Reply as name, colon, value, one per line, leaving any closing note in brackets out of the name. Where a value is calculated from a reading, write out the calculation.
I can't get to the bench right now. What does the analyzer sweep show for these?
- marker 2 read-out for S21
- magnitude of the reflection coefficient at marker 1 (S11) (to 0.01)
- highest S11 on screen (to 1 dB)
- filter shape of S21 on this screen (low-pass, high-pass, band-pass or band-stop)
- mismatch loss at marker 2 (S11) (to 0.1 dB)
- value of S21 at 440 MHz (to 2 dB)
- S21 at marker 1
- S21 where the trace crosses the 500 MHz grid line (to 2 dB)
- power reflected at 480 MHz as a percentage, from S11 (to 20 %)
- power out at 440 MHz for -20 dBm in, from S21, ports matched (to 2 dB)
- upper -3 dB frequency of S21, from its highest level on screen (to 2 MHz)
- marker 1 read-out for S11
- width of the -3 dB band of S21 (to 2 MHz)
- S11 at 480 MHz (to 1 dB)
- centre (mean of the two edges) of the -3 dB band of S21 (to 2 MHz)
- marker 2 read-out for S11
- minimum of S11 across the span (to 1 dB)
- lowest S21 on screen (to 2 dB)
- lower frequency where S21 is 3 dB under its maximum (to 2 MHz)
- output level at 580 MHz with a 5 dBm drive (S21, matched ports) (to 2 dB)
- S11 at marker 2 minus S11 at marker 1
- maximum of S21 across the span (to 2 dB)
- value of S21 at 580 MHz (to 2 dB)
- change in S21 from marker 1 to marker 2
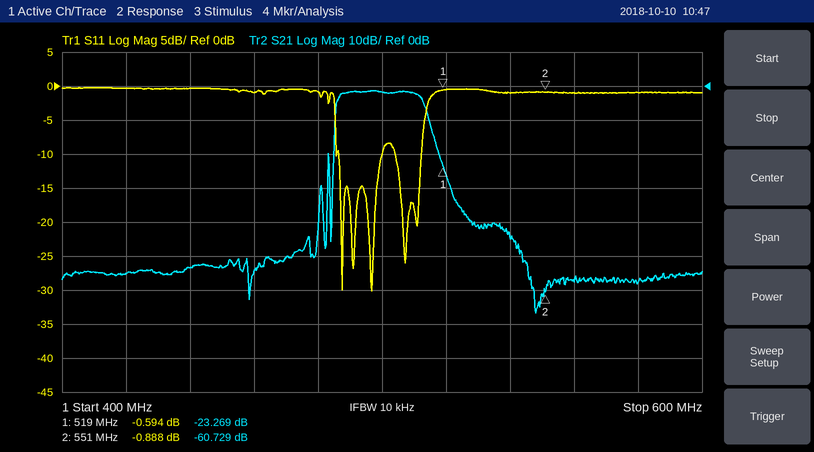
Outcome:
marker 2 read-out for S21: -60.729 dB
magnitude of the reflection coefficient at marker 1 (S11): 10^(-0.594/20) ≈ 0.93
highest S11 on screen: 0 dB
filter shape of S21 on this screen: band-pass
mismatch loss at marker 2 (S11): −10 log10(1 − 10^(-0.888/10)) ≈ 7.3 dB
value of S21 at 440 MHz: -54 dB
S21 at marker 1: -23.269 dB
S21 where the trace crosses the 500 MHz grid line: -2 dB
power reflected at 480 MHz as a percentage, from S11: 10^(-1/10) ≈ 79.4 %, so 80 % to the nearest 20 %
power out at 440 MHz for -20 dBm in, from S21, ports matched: -20 dBm + (-54 dB) = -74 dBm
upper -3 dB frequency of S21, from its highest level on screen: 512 MHz
marker 1 read-out for S11: -0.594 dB
width of the -3 dB band of S21: 512 MHz − 486 MHz = 26 MHz
S11 at 480 MHz: -1 dB
centre (mean of the two edges) of the -3 dB band of S21: 500 MHz
marker 2 read-out for S11: -0.888 dB
minimum of S11 across the span: -30 dB
lowest S21 on screen: -66 dB
lower frequency where S21 is 3 dB under its maximum: 486 MHz
output level at 580 MHz with a 5 dBm drive (S21, matched ports): 5 dBm + (-58 dB) = -52 dBm
S11 at marker 2 minus S11 at marker 1: -0.888 − (-0.594) = -0.294 dB
maximum of S21 across the span: -2 dB
value of S21 at 580 MHz: -58 dB
change in S21 from marker 1 to marker 2: -60.729 − (-23.269) = -37.460 dB
